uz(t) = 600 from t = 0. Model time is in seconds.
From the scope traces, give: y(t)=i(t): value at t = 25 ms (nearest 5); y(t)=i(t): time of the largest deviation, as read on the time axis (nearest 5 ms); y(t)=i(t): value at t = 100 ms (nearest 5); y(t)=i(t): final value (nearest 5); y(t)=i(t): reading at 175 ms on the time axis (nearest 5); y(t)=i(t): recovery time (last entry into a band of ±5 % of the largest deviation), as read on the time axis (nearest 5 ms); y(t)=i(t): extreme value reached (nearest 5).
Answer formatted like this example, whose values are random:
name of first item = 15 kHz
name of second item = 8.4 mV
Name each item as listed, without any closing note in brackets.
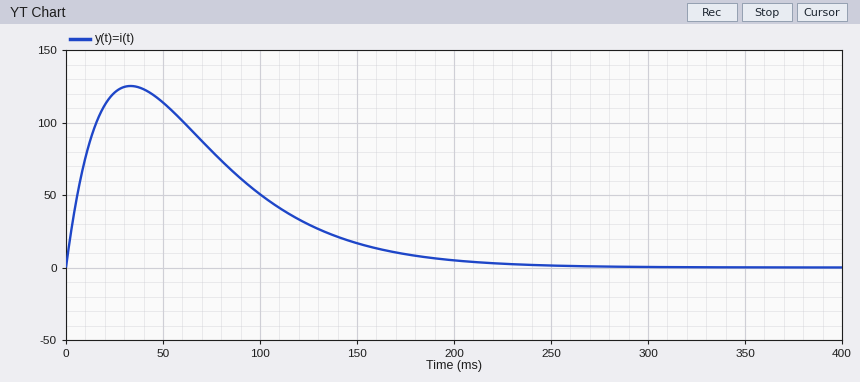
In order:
y(t)=i(t): value at t = 25 ms = 120
y(t)=i(t): time of the largest deviation, as read on the time axis = 35 ms
y(t)=i(t): value at t = 100 ms = 50
y(t)=i(t): final value = 0
y(t)=i(t): reading at 175 ms on the time axis = 10
y(t)=i(t): recovery time (last entry into a band of ±5 % of the largest deviation), as read on the time axis = 190 ms
y(t)=i(t): extreme value reached = 125
